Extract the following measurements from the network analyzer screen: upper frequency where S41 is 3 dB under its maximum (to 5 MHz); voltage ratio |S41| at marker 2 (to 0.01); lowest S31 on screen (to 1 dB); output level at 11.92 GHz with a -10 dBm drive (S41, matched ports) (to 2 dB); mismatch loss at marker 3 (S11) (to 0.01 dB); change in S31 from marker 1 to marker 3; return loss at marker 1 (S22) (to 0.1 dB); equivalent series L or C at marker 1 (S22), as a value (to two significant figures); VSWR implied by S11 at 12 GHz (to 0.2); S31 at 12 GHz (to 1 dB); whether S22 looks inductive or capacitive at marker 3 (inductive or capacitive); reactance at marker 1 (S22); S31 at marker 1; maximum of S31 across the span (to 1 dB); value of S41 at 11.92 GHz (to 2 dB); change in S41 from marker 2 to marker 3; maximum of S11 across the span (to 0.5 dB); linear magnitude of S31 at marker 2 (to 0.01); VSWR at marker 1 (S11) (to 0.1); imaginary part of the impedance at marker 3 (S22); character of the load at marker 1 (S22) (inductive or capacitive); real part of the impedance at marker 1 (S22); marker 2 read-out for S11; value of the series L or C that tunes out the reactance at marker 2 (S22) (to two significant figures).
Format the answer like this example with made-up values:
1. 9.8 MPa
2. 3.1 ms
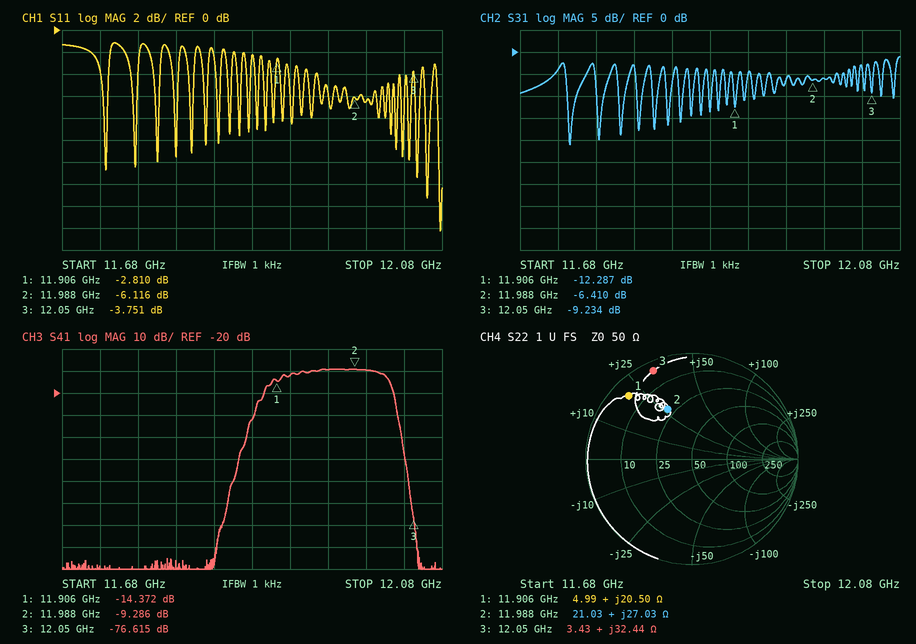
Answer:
1. 12.020 GHz
2. 0.34
3. -21 dB
4. -22 dBm
5. 2.38 dB
6. 3.053 dB
7. 1.5 dB
8. 270 pH
9. 2.8
10. -6 dB
11. inductive
12. +20.50 Ω
13. -12.287 dB
14. -1 dB
15. -12 dB
16. -67.329 dB
17. -1.0 dB
18. 0.48
19. 6.2
20. +32.44 Ω
21. inductive
22. 4.99 Ω
23. -6.116 dB
24. 490 fF
